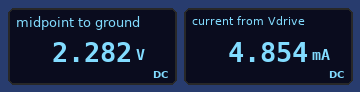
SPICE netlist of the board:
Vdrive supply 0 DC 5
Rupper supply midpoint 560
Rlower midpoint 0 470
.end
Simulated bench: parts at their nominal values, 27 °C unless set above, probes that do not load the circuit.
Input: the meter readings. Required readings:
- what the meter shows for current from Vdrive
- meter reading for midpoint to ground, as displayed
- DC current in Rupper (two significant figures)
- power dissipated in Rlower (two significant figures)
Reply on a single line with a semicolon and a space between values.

4.854 mA; 2.282 V; 4.9 mA; 11 mW
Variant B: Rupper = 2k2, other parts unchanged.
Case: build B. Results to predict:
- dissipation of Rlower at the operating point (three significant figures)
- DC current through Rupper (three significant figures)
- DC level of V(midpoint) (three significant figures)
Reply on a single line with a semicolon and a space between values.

1.65 mW; 1.87 mA; 880 mV
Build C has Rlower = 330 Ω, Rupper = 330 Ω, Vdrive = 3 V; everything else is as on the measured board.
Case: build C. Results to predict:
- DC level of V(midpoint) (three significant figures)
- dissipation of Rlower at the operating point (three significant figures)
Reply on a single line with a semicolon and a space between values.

1.50 V; 6.82 mW
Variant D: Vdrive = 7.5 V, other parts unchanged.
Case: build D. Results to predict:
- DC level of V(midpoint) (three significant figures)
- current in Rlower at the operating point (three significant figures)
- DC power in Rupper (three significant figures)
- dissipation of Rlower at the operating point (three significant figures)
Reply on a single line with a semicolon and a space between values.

3.42 V; 7.28 mA; 29.7 mW; 24.9 mW
